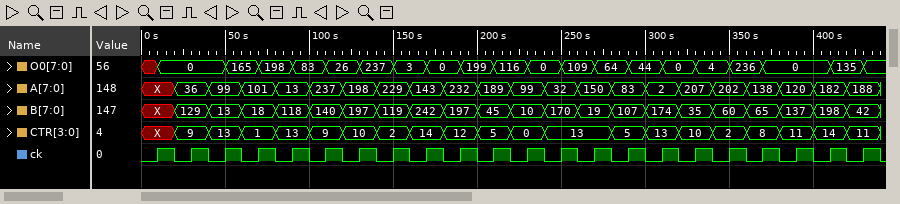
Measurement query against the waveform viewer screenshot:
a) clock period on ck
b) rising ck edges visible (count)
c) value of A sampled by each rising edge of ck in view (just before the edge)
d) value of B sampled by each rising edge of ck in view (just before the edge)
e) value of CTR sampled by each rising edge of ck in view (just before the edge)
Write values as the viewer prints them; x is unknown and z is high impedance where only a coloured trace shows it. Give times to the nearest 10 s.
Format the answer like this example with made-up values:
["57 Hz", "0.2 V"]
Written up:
["20 s", "22", "X, 36, 99, 101, 13, 237, 198, 229, 143, 232, 189, 99, 32, 150, 83, 2, 207, 202, 138, 120, 182, 188", "X, 129, 13, 18, 118, 140, 197, 119, 242, 197, 45, 10, 170, 19, 107, 174, 35, 60, 65, 137, 198, 42", "X, 9, 13, 1, 13, 9, 10, 2, 14, 12, 5, 0, 13, 13, 5, 13, 10, 2, 8, 11, 14, 11"]
